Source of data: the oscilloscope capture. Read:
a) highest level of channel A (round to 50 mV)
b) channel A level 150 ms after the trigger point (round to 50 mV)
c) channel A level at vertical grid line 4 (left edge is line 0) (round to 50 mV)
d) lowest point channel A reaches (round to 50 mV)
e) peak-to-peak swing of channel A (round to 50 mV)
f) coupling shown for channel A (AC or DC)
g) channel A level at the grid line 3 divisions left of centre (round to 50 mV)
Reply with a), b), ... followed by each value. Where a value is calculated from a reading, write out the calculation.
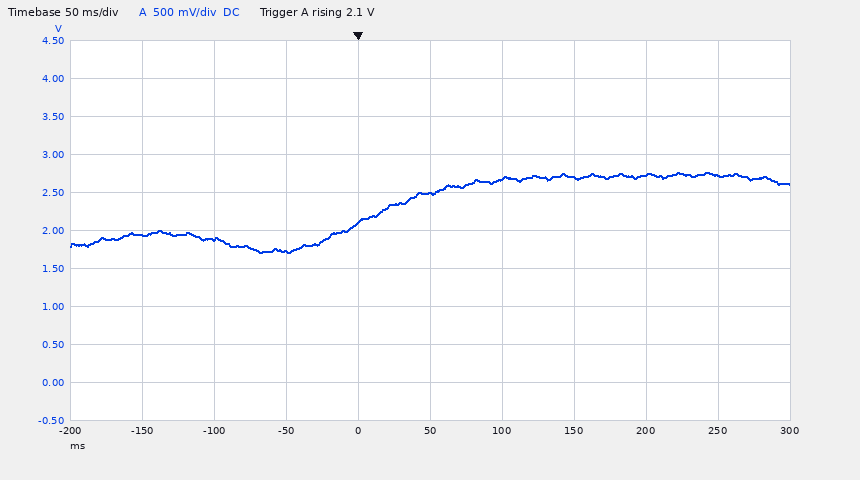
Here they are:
a) 2.75 V
b) 2.70 V
c) 2.10 V
d) 1.70 V
e) 2.75 V − (1.70 V) = 1.05 V
f) DC
g) 1.90 V
